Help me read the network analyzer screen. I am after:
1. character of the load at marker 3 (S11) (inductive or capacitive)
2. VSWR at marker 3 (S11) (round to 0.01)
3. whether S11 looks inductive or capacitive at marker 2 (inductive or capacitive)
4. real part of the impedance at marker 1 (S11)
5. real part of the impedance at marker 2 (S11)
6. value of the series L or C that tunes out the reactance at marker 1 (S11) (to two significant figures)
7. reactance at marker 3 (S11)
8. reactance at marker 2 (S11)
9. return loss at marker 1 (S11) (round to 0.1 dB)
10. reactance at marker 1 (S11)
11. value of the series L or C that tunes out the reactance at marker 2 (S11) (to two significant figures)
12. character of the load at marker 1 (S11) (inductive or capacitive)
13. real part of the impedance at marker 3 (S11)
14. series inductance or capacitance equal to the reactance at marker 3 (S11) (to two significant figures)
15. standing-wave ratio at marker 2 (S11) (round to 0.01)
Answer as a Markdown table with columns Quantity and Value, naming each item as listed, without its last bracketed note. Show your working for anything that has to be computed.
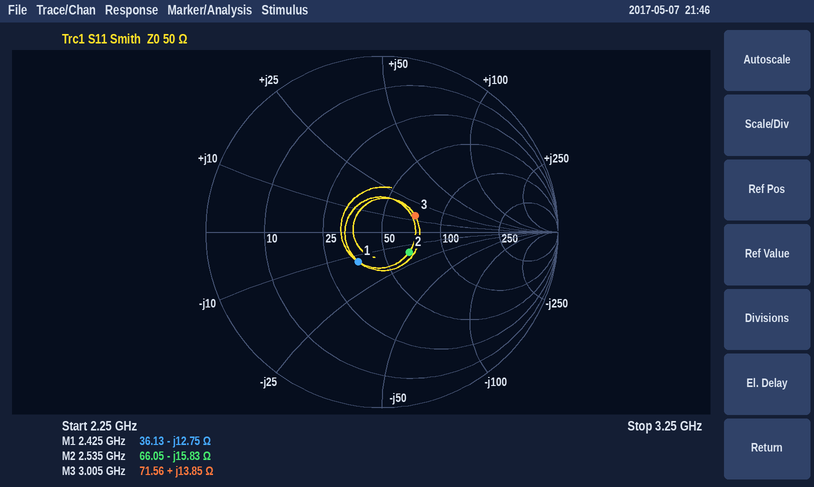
| Quantity | Value |
|---|---|
| character of the load at marker 3 (S11) | inductive |
| VSWR at marker 3 (S11) | 1.53 |
| whether S11 looks inductive or capacitive at marker 2 | capacitive |
| real part of the impedance at marker 1 | 36.13 Ω |
| real part of the impedance at marker 2 | 66.05 Ω |
| value of the series L or C that tunes out the reactance at marker 1 (S11) | L = 12.75 Ω/(2π × 2.425 GHz) ≈ 837 pH, so 840 pH to two significant figures |
| reactance at marker 3 | +13.85 Ω |
| reactance at marker 2 | -15.83 Ω |
| return loss at marker 1 (S11) | 13.3 dB |
| reactance at marker 1 | -12.75 Ω |
| value of the series L or C that tunes out the reactance at marker 2 (S11) | L = 15.83 Ω/(2π × 2.535 GHz) ≈ 994 pH, so 990 pH to two significant figures |
| character of the load at marker 1 (S11) | capacitive |
| real part of the impedance at marker 3 | 71.56 Ω |
| series inductance or capacitance equal to the reactance at marker 3 (S11) | L = 13.85 Ω/(2π × 3.005 GHz) ≈ 734 pH, so 730 pH to two significant figures |
| standing-wave ratio at marker 2 (S11) | 1.48 |
